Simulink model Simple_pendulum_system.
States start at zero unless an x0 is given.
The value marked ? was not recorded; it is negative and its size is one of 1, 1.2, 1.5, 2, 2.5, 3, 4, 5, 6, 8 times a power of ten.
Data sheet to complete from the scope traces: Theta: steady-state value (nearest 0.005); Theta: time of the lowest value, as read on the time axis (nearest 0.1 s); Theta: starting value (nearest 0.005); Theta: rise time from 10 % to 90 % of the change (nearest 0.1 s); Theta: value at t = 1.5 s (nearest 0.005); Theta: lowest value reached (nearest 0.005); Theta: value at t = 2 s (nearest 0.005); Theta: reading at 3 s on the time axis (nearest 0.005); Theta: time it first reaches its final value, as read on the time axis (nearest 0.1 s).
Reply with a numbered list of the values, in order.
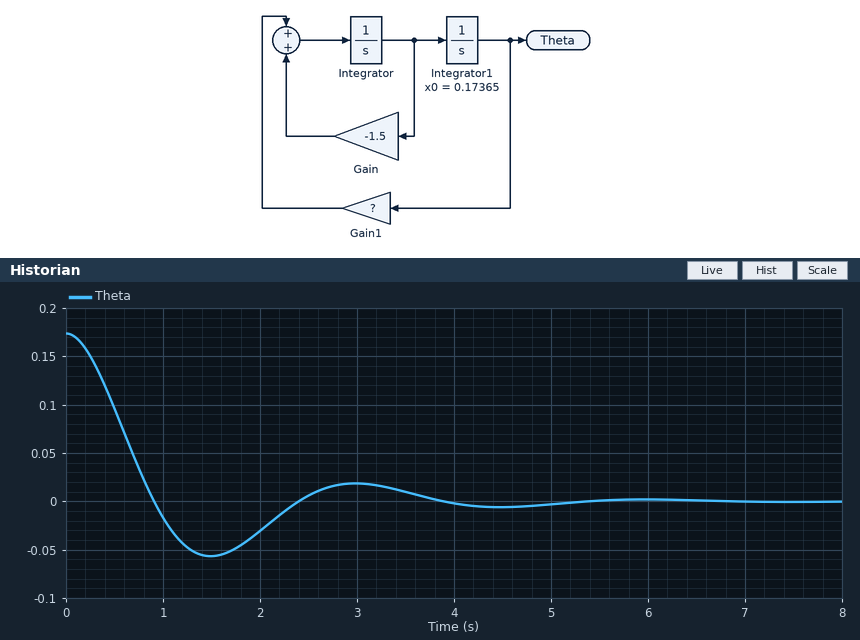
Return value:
1. 0.000
2. 1.5 s
3. 0.175
4. 0.6 s
5. -0.055
6. -0.055
7. -0.030
8. 0.020
9. 0.9 s
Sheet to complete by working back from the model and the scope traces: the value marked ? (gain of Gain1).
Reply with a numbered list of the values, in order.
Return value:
1. -5
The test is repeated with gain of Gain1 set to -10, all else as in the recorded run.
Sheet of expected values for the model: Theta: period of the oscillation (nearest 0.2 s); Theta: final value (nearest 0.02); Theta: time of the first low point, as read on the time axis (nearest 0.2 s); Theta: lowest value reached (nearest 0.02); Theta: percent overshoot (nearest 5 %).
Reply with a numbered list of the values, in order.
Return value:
1. 2.0 s
2. 0.00
3. 1.0 s
4. -0.08
5. 45 %
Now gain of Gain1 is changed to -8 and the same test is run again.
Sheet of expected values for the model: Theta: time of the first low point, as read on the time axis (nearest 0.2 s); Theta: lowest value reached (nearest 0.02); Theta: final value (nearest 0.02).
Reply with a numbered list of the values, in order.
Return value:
1. 1.2 s
2. -0.08
3. 0.00
